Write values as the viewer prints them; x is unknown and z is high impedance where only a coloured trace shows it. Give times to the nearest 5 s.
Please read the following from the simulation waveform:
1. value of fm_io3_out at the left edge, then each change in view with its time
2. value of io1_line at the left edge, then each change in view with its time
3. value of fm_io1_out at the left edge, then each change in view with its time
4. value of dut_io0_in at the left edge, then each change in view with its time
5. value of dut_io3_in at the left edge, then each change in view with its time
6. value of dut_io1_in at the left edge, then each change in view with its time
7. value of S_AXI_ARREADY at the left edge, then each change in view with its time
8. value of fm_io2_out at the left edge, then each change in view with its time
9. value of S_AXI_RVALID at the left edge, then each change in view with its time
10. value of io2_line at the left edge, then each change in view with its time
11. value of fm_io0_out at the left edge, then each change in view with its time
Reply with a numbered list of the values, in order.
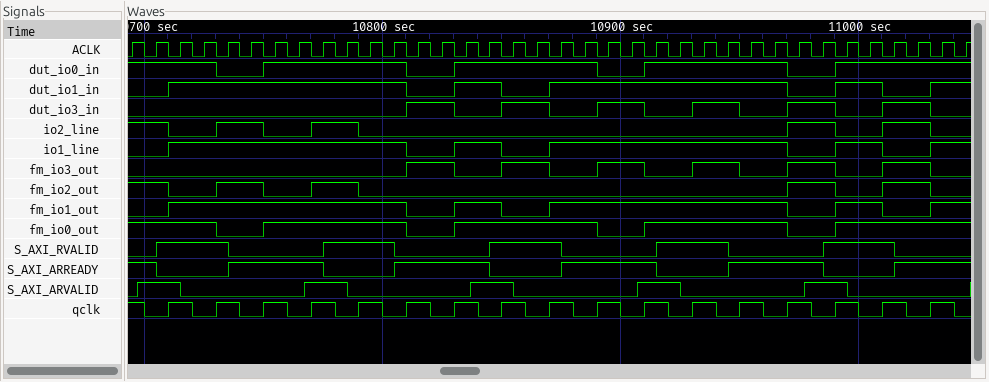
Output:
1. 0, 1 at 10810 s, 0 at 10830 s, 1 at 10850 s, 0 at 10870 s, 1 at 10890 s, 0 at 10910 s, 1 at 10930 s, 0 at 10950 s, 1 at 10970 s, 0 at 10990 s, 1 at 11010 s, 0 at 11030 s
2. 0, 1 at 10710 s, 0 at 10810 s, 1 at 10830 s, 0 at 10850 s, 1 at 10870 s, 0 at 10970 s, 1 at 10990 s, 0 at 11010 s, 1 at 11030 s
3. 0, 1 at 10710 s, 0 at 10810 s, 1 at 10830 s, 0 at 10850 s, 1 at 10870 s, 0 at 10970 s, 1 at 10990 s, 0 at 11010 s, 1 at 11030 s
4. 1, 0 at 10730 s, 1 at 10750 s, 0 at 10810 s, 1 at 10830 s, 0 at 10890 s, 1 at 10910 s, 0 at 10970 s, 1 at 10990 s
5. 0, 1 at 10810 s, 0 at 10830 s, 1 at 10850 s, 0 at 10870 s, 1 at 10890 s, 0 at 10910 s, 1 at 10930 s, 0 at 10950 s, 1 at 10970 s, 0 at 10990 s, 1 at 11010 s, 0 at 11030 s
6. 0, 1 at 10710 s, 0 at 10810 s, 1 at 10830 s, 0 at 10850 s, 1 at 10870 s, 0 at 10970 s, 1 at 10990 s, 0 at 11010 s, 1 at 11030 s
7. 1, 0 at 10705 s, 1 at 10735 s, 0 at 10775 s, 1 at 10805 s, 0 at 10845 s, 1 at 10875 s, 0 at 10915 s, 1 at 10945 s, 0 at 10985 s, 1 at 11015 s
8. 1, 0 at 10710 s, 1 at 10730 s, 0 at 10750 s, 1 at 10770 s, 0 at 10790 s, 1 at 10970 s, 0 at 10990 s, 1 at 11010 s, 0 at 11030 s
9. 0, 1 at 10705 s, 0 at 10735 s, 1 at 10775 s, 0 at 10805 s, 1 at 10845 s, 0 at 10875 s, 1 at 10915 s, 0 at 10945 s, 1 at 10985 s, 0 at 11015 s
10. 1, 0 at 10710 s, 1 at 10730 s, 0 at 10750 s, 1 at 10770 s, 0 at 10790 s, 1 at 10970 s, 0 at 10990 s, 1 at 11010 s, 0 at 11030 s
11. 1, 0 at 10730 s, 1 at 10750 s, 0 at 10810 s, 1 at 10830 s, 0 at 10890 s, 1 at 10910 s, 0 at 10970 s, 1 at 10990 s
